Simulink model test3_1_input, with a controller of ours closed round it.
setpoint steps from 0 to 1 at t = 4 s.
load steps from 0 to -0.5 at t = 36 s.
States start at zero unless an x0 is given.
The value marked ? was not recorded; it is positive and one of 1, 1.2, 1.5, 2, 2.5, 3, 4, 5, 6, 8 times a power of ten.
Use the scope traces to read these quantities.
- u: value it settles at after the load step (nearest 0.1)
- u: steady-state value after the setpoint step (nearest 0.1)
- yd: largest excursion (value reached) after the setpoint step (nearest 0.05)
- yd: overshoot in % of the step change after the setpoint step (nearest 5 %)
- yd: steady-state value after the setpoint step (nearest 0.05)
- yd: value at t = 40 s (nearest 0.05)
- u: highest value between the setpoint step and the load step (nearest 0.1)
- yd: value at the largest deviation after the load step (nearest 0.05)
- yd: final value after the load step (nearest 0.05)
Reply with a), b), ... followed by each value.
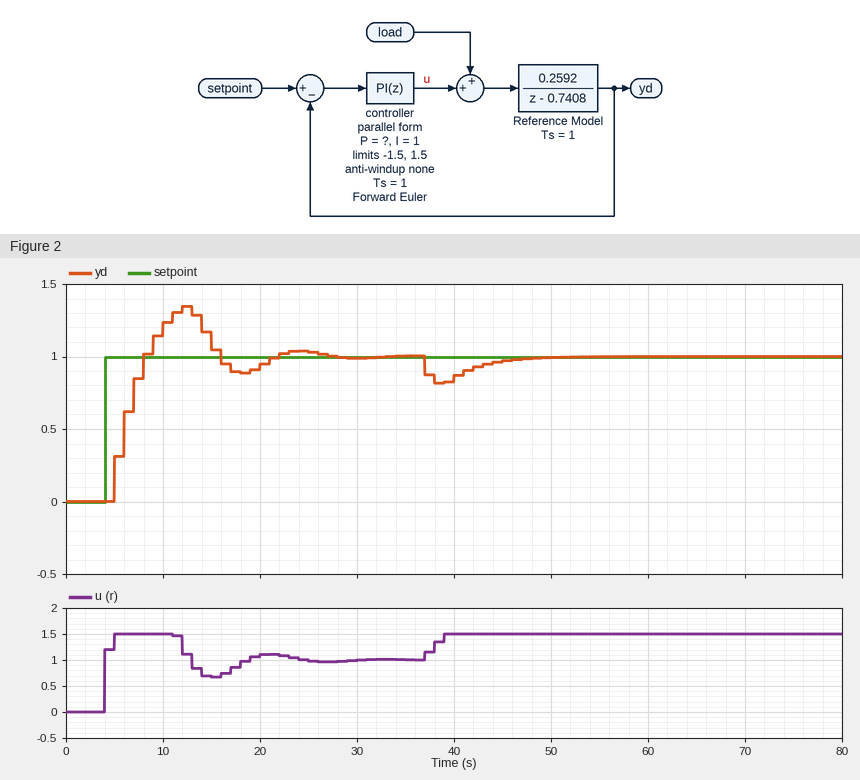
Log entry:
a) 1.5
b) 1.0
c) 1.35
d) 35 %
e) 1.00
f) 0.85
g) 1.5
h) 0.80
i) 1.00
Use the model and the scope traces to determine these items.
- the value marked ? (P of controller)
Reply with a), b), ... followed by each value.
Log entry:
a) 1.2
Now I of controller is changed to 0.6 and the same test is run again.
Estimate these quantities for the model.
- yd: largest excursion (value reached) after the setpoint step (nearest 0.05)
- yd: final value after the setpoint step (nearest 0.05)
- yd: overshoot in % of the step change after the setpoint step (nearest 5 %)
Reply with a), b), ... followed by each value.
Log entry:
a) 1.15
b) 1.00
c) 15 %
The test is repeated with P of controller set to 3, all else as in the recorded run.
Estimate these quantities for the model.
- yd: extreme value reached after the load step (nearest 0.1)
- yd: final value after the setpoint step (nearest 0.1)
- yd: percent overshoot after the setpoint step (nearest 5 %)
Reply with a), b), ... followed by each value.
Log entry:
a) 0.9
b) 1.0
c) 25 %
